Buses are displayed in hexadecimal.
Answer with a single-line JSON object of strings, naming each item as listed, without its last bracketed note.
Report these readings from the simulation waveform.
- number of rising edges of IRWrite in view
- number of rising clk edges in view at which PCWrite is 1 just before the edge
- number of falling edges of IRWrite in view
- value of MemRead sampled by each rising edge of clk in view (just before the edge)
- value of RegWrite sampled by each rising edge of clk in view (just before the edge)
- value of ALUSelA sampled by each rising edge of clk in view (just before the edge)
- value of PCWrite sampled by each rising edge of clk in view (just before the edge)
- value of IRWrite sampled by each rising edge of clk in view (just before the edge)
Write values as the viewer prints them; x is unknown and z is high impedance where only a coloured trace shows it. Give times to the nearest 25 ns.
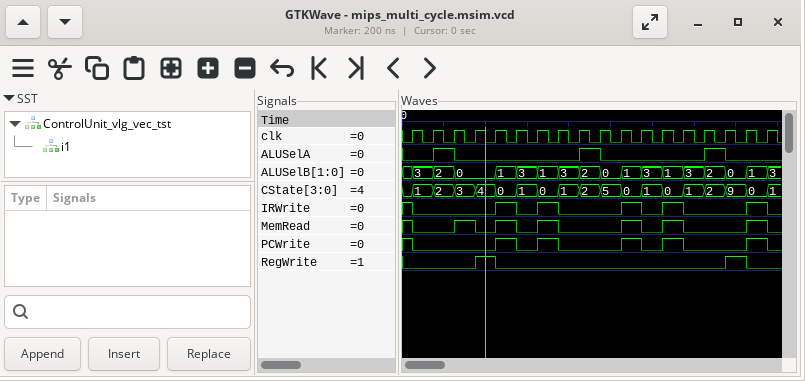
{"number of rising edges of IRWrite in view": "5", "number of rising clk edges in view at which PCWrite is 1 just before the edge": "6", "number of falling edges of IRWrite in view": "6", "value of MemRead sampled by each rising edge of clk in view": "1 0 0 1 0 1 0 1 0 0 0 1 0 1 0 0 0 1", "value of RegWrite sampled by each rising edge of clk in view": "0 0 0 0 1 0 0 0 0 0 0 0 0 0 0 0 1 0", "value of ALUSelA sampled by each rising edge of clk in view": "0 0 1 0 0 0 0 0 0 1 0 0 0 0 0 1 0 0", "value of PCWrite sampled by each rising edge of clk in view": "1 0 0 0 0 1 0 1 0 0 0 1 0 1 0 0 0 1", "value of IRWrite sampled by each rising edge of clk in view": "1 0 0 0 0 1 0 1 0 0 0 1 0 1 0 0 0 1"}
